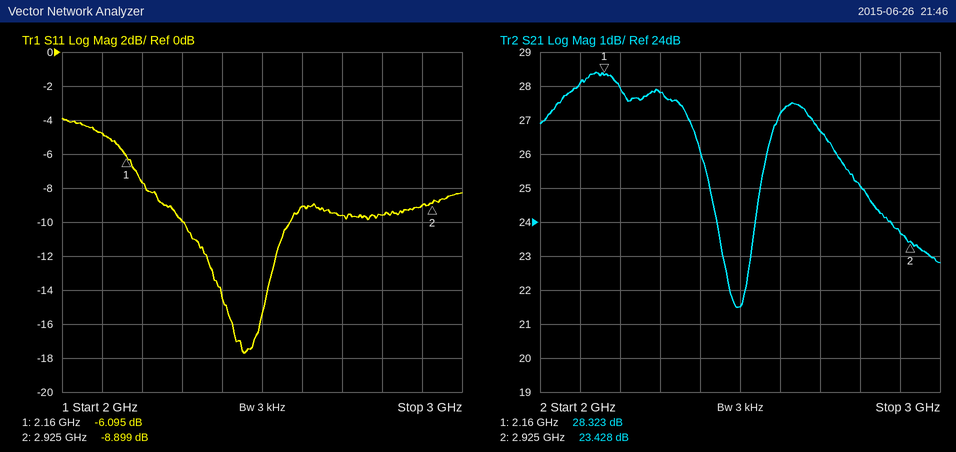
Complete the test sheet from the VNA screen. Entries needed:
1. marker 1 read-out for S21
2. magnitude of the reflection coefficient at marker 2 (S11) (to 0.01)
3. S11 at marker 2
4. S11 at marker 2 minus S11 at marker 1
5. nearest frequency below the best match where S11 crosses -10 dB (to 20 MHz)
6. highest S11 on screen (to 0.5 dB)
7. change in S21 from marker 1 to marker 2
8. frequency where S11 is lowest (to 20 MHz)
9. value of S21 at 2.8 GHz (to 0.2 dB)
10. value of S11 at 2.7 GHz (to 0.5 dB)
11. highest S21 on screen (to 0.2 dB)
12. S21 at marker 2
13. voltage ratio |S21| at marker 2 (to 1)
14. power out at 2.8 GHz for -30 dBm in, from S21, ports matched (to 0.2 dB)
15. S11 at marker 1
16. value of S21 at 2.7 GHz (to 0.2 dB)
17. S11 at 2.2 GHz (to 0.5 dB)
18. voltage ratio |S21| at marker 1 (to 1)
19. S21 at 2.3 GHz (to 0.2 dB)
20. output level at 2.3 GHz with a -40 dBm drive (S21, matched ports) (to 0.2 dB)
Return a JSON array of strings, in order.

["28.323 dB", "0.36", "-8.899 dB", "-2.804 dB", "2.30 GHz", "-4.0 dB", "-4.895 dB", "2.46 GHz", "25.0 dB", "-9.5 dB", "28.4 dB", "23.428 dB", "15", "-5.0 dBm", "-6.095 dB", "26.6 dB", "-7.5 dB", "26", "27.8 dB", "-12.2 dBm"]
